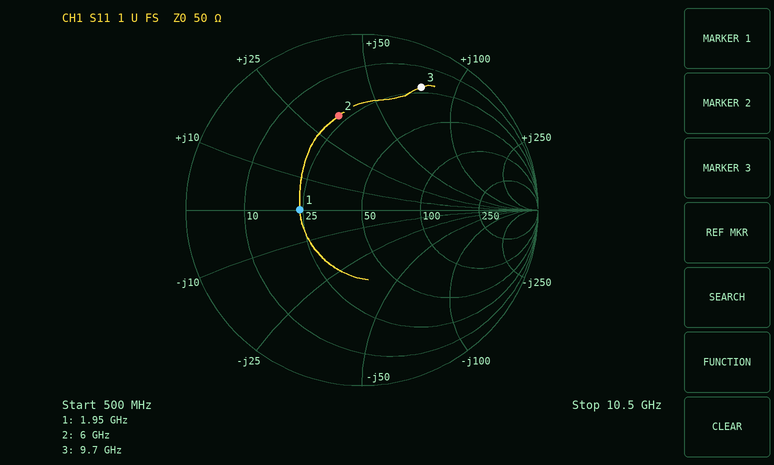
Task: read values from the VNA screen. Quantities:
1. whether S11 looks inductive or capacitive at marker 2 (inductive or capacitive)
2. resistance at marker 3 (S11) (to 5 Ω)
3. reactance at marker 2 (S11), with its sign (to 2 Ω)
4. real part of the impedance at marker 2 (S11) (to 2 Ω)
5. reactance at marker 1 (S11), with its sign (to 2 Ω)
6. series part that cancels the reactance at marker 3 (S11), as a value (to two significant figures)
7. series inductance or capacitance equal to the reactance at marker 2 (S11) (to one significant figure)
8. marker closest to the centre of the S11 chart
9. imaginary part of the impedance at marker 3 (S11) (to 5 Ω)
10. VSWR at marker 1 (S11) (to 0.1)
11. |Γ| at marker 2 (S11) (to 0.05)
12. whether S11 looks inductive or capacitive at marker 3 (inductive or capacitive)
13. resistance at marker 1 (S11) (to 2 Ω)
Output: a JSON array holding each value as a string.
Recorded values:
["inductive", "20 Ω", "+34 Ω", "22 Ω", "0 Ω", "220 fF", "900 pH", "marker 1", "+75 Ω", "2.1", "0.55", "inductive", "24 Ω"]
